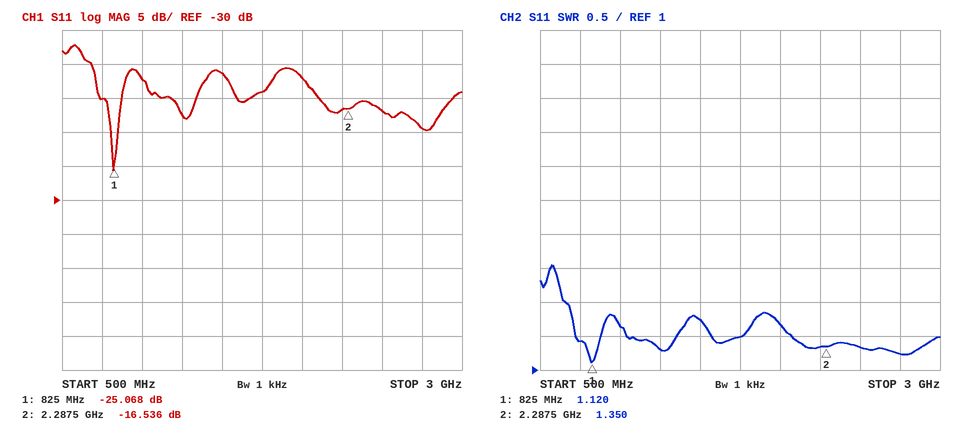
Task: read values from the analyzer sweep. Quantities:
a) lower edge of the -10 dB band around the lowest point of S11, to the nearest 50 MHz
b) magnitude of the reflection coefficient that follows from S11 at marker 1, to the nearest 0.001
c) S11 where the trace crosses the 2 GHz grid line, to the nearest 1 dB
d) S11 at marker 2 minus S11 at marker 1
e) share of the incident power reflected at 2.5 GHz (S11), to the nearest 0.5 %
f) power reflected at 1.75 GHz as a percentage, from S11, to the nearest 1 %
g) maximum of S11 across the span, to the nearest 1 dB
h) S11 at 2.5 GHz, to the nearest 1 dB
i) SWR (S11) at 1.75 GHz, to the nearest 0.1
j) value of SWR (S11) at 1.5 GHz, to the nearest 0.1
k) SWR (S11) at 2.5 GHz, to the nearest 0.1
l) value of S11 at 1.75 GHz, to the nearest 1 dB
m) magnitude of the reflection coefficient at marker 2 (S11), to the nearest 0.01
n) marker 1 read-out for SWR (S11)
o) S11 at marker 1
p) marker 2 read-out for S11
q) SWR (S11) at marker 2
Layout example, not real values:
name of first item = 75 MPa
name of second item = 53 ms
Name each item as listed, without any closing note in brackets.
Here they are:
lower edge of the -10 dB band around the lowest point of S11, to the nearest 50 MHz = 700 MHz
magnitude of the reflection coefficient that follows from S11 at marker 1, to the nearest 0.001 = 0.056
S11 where the trace crosses the 2 GHz grid line, to the nearest 1 dB = -12 dB
S11 at marker 2 minus S11 at marker 1 = 8.532 dB
share of the incident power reflected at 2.5 GHz (S11), to the nearest 0.5 % = 2.0 %
power reflected at 1.75 GHz as a percentage, from S11, to the nearest 1 % = 4 %
maximum of S11 across the span, to the nearest 1 dB = -7 dB
S11 at 2.5 GHz, to the nearest 1 dB = -17 dB
SWR (S11) at 1.75 GHz, to the nearest 0.1 = 1.5
value of SWR (S11) at 1.5 GHz, to the nearest 0.1 = 1.7
SWR (S11) at 2.5 GHz, to the nearest 0.1 = 1.3
value of S11 at 1.75 GHz, to the nearest 1 dB = -14 dB
magnitude of the reflection coefficient at marker 2 (S11), to the nearest 0.01 = 0.15
marker 1 read-out for SWR = 1.120
S11 at marker 1 = -25.068 dB
marker 2 read-out for S11 = -16.536 dB
SWR (S11) at marker 2 = 1.350
